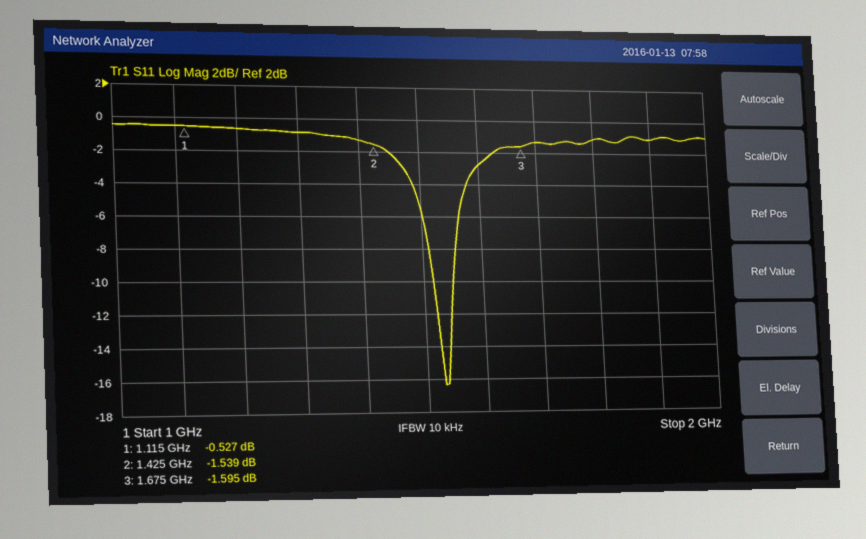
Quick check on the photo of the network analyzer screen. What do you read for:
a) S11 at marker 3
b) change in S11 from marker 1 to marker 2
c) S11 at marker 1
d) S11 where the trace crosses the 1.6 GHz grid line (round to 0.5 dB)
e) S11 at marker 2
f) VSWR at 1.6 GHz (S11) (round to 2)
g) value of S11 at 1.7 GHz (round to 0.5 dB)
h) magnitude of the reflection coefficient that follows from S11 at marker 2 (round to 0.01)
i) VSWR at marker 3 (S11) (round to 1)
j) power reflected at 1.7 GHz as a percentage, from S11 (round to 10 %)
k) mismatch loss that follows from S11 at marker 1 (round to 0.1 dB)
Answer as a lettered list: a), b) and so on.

a) -1.595 dB
b) -1.012 dB
c) -0.527 dB
d) -3.0 dB
e) -1.539 dB
f) 6
g) -1.5 dB
h) 0.84
i) 11
j) 70 %
k) 9.4 dB
